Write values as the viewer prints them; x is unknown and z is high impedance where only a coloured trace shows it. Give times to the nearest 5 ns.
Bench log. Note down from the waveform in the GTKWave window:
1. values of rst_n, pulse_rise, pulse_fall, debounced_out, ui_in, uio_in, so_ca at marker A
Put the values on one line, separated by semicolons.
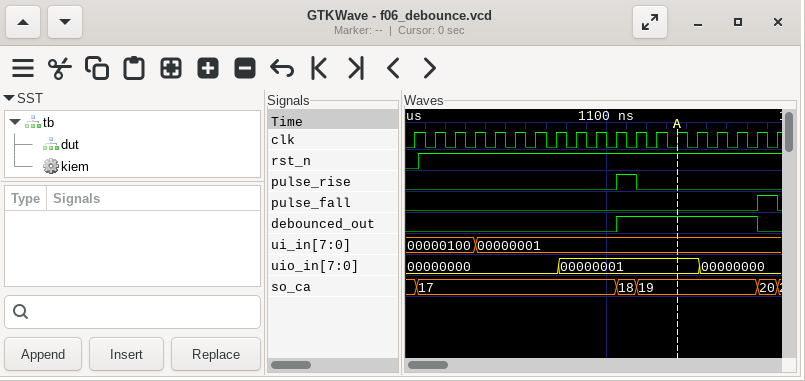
rst_n=1, pulse_rise=0, pulse_fall=0, debounced_out=1, ui_in=00000001, uio_in=00000001, so_ca=19
